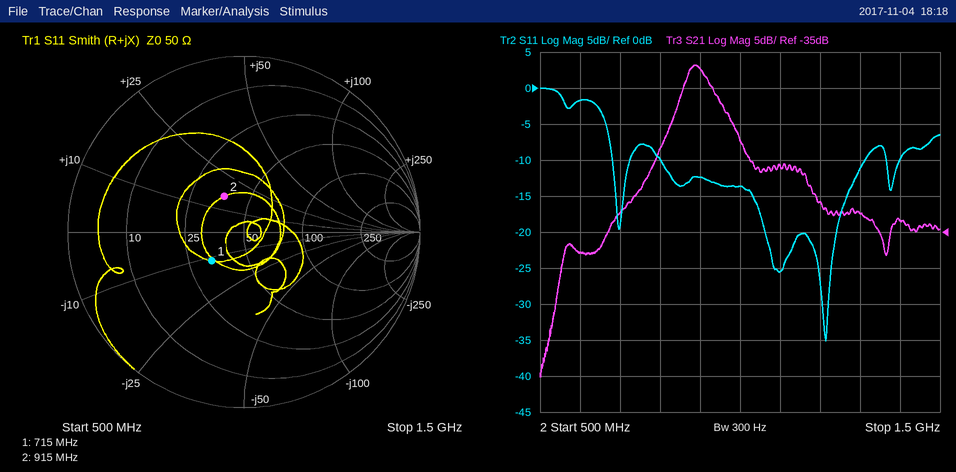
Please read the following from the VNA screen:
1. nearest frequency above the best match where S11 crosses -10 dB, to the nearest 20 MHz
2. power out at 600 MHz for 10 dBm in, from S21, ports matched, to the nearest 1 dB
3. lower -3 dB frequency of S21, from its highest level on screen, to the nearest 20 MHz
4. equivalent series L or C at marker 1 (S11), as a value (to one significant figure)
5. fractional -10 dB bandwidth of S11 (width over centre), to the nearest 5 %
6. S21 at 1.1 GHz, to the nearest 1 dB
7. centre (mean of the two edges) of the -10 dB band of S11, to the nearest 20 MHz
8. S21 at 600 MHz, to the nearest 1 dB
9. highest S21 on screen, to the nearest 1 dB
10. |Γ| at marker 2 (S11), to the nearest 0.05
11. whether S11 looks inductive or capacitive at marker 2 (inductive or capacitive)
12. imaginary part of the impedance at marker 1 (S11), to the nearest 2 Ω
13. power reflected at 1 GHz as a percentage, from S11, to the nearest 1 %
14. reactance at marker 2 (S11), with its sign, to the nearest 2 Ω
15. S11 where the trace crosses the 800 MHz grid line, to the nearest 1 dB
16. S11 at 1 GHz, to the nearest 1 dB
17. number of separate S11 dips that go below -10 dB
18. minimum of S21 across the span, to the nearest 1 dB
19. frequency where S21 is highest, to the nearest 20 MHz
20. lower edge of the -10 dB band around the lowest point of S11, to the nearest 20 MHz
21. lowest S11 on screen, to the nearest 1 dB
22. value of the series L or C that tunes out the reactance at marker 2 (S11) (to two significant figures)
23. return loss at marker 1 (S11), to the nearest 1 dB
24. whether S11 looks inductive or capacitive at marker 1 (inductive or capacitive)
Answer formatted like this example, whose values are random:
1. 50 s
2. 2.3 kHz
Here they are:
1. 1.32 GHz
2. -28 dBm
3. 860 MHz
4. 20 pF
5. 50 %
6. -26 dB
7. 1.06 GHz
8. -38 dB
9. -12 dB
10. 0.25
11. inductive
12. -12 Ω
13. 4 %
14. +16 Ω
15. -10 dB
16. -14 dB
17. 4
18. -55 dB
19. 880 MHz
20. 800 MHz
21. -35 dB
22. 11 pF
23. 12 dB
24. capacitive
